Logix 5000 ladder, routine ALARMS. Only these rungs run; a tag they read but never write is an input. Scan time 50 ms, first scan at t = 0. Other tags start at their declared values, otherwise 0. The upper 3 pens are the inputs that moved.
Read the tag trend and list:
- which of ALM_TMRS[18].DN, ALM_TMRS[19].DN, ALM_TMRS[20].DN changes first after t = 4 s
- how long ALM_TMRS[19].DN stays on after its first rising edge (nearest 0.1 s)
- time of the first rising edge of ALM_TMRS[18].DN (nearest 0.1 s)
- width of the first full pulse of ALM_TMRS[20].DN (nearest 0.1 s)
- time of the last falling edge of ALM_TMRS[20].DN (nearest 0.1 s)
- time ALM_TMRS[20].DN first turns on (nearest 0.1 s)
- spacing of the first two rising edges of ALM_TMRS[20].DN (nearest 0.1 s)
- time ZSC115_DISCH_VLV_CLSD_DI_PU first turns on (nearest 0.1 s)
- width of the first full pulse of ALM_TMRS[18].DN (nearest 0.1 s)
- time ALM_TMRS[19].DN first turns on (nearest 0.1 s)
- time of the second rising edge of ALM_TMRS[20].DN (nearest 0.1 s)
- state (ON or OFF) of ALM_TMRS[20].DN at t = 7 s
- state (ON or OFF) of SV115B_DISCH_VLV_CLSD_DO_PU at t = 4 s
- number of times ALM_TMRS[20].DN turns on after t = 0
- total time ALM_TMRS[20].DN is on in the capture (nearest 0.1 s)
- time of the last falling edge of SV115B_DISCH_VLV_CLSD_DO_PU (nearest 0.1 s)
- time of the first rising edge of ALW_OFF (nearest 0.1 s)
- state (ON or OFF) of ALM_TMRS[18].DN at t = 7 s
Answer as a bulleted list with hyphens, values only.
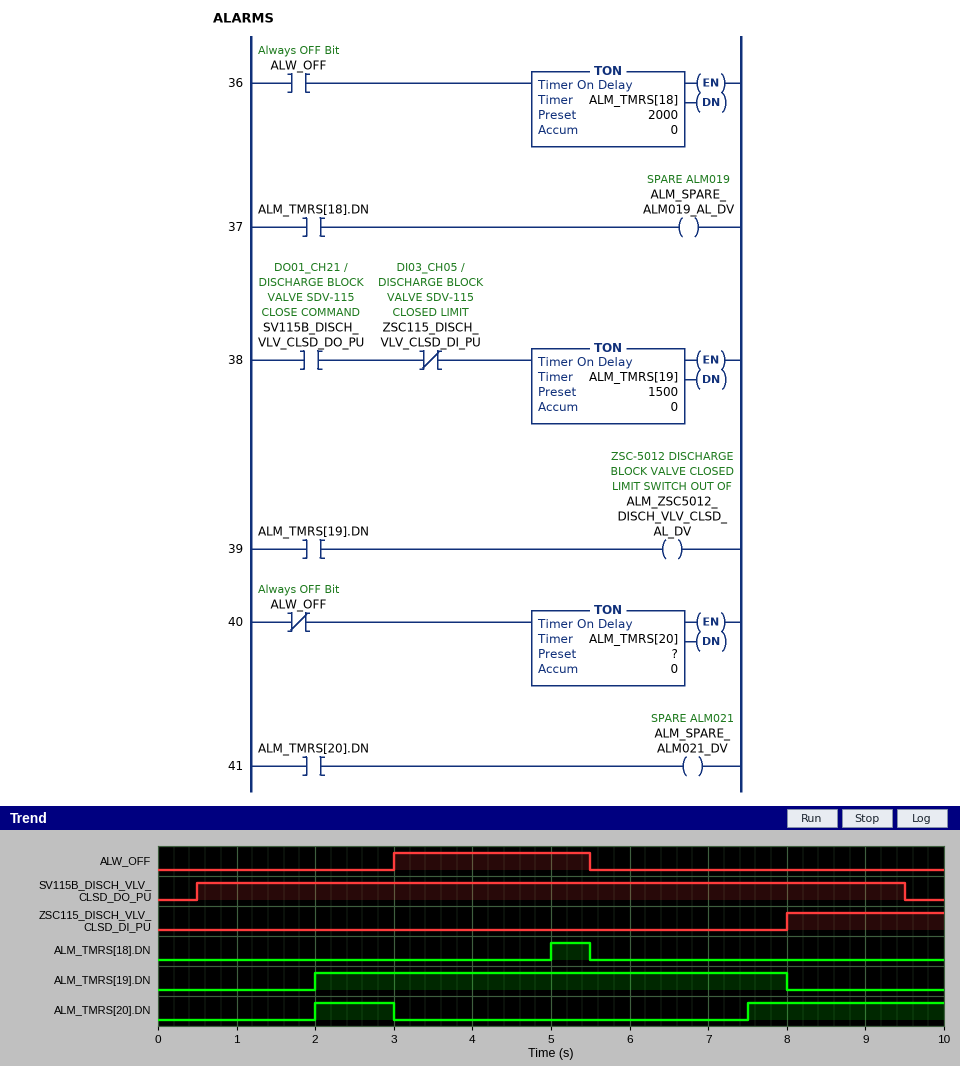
- ALM_TMRS[18].DN
- 6.0 s
- 5.0 s
- 1.0 s
- 3.0 s
- 2.0 s
- 5.5 s
- 8.0 s
- 0.5 s
- 2.0 s
- 7.5 s
- OFF
- ON
- 2
- 3.5 s
- 9.5 s
- 3.0 s
- OFF
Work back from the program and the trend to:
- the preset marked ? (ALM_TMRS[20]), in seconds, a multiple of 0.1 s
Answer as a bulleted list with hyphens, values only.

- 2.0 s
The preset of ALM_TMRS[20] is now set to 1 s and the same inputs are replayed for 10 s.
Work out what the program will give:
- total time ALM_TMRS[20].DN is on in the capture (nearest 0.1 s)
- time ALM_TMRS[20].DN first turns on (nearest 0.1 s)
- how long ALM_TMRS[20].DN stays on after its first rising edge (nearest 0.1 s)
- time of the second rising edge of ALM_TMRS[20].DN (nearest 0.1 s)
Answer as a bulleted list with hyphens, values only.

- 5.5 s
- 1.0 s
- 2.0 s
- 6.5 s
